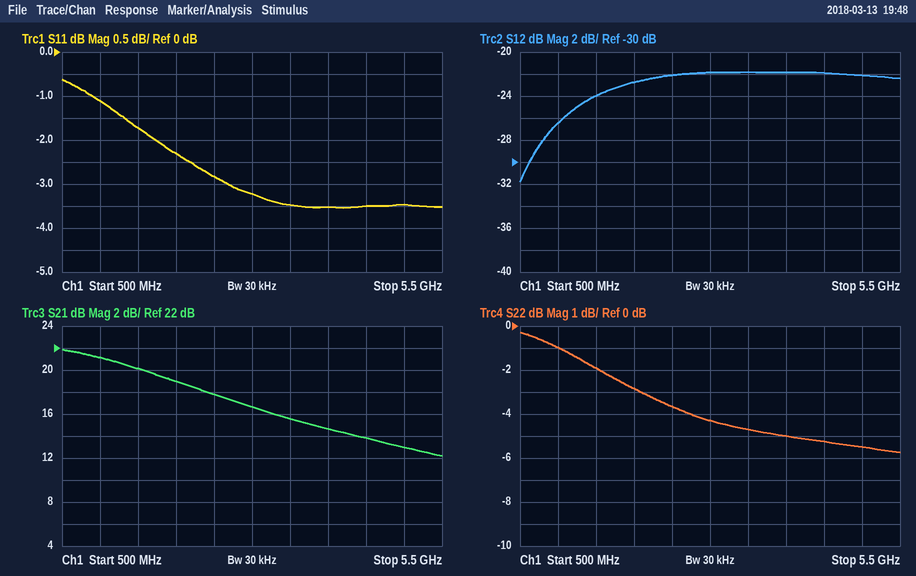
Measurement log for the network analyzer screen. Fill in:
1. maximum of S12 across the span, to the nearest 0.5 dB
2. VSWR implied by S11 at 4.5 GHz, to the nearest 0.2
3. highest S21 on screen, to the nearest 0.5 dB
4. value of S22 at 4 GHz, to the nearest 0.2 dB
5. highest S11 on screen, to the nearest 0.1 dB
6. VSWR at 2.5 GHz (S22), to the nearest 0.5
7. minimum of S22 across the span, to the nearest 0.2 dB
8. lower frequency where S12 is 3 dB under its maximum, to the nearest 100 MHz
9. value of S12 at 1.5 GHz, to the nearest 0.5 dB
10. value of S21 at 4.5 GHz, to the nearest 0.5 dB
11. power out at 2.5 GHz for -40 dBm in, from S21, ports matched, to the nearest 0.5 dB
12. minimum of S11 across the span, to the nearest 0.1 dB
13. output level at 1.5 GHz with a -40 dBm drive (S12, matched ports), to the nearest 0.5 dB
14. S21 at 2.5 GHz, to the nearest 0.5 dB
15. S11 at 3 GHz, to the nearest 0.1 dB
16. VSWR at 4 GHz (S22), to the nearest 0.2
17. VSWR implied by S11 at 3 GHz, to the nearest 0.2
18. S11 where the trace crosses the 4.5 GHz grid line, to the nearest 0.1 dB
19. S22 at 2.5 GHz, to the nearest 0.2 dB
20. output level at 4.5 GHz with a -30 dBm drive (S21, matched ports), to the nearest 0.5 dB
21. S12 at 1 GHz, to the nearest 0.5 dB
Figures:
-22.0 dB
5.0
22.0 dB
-5.0 dB
-0.6 dB
5.0
-5.8 dB
1.3 GHz
-24.0 dB
14.0 dB
-22.0 dBm
-3.5 dB
-64.0 dBm
18.0 dB
-3.2 dB
3.6
5.4
-3.5 dB
-3.6 dB
-16.0 dBm
-26.5 dB
